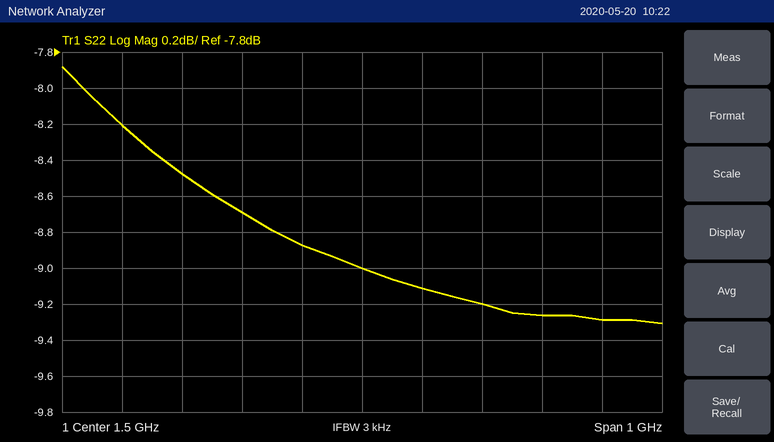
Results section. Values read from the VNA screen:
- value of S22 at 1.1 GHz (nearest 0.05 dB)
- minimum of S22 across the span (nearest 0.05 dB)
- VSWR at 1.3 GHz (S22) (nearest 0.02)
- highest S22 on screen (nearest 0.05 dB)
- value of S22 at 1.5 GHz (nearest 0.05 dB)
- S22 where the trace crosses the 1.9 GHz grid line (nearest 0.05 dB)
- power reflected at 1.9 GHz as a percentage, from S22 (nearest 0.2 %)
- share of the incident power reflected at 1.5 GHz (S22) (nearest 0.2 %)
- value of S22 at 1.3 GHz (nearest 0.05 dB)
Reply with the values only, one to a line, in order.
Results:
-8.20 dB
-9.30 dB
2.16
-7.90 dB
-9.00 dB
-9.30 dB
11.8 %
12.6 %
-8.70 dB
